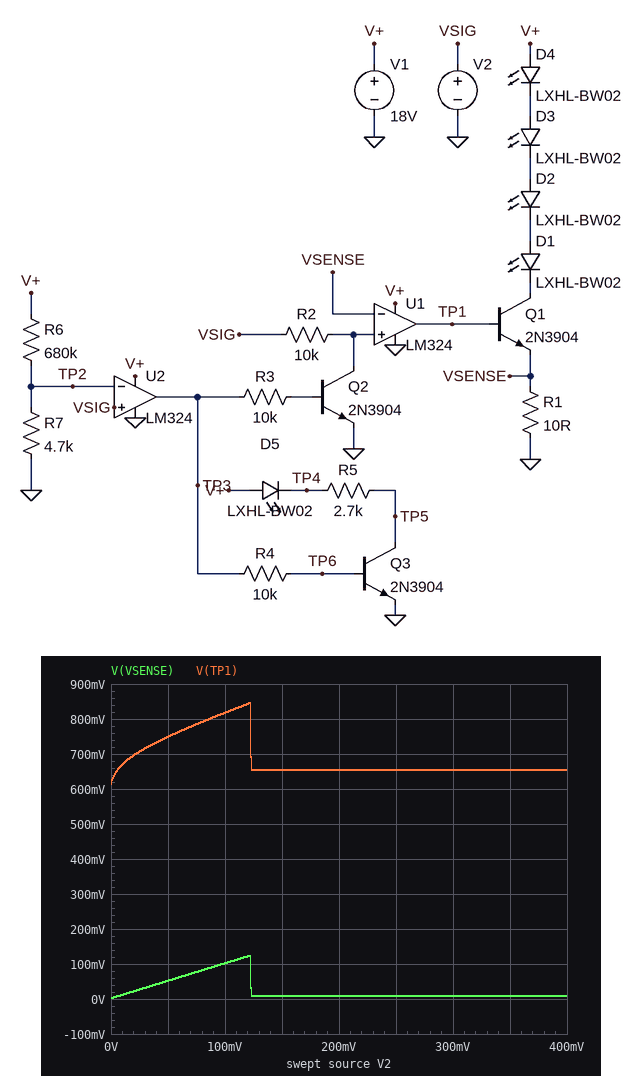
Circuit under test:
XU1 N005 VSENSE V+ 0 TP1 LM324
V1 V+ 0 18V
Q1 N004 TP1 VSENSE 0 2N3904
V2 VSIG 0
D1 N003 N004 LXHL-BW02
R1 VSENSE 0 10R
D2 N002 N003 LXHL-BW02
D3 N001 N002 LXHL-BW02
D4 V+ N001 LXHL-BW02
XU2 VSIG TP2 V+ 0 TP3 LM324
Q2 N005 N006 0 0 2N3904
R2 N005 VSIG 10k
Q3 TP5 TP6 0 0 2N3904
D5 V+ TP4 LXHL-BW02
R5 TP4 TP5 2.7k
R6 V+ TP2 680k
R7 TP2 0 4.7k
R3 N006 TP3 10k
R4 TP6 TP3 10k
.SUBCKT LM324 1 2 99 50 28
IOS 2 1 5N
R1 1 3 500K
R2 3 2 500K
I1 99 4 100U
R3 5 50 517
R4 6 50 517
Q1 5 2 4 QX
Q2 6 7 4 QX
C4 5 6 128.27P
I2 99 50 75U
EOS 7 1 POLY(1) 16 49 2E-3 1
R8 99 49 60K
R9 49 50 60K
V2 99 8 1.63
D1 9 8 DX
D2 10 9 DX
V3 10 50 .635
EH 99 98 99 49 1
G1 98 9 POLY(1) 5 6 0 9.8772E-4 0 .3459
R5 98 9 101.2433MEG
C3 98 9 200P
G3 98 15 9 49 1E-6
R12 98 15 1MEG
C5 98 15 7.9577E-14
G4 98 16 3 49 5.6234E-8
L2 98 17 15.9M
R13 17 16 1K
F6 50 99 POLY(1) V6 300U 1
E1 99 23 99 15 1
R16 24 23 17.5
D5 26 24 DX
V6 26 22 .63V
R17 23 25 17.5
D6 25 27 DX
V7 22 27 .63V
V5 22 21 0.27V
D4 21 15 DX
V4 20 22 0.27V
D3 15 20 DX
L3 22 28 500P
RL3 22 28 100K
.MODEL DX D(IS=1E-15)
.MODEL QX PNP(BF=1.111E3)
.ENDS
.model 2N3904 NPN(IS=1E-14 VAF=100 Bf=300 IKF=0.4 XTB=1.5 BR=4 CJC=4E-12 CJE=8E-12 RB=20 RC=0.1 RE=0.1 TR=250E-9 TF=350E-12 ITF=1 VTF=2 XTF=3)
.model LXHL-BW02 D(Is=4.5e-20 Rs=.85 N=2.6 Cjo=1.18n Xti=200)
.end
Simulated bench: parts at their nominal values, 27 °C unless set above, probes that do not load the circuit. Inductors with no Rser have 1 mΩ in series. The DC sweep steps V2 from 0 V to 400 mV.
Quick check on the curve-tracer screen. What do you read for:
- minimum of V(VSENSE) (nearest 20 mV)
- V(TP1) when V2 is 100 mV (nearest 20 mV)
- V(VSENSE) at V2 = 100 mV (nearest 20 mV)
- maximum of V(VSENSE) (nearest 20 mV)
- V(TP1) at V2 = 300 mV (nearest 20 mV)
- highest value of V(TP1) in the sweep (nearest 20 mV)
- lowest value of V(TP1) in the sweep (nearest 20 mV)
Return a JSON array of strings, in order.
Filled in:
["0 V", "820 mV", "100 mV", "120 mV", "660 mV", "840 mV", "620 mV"]
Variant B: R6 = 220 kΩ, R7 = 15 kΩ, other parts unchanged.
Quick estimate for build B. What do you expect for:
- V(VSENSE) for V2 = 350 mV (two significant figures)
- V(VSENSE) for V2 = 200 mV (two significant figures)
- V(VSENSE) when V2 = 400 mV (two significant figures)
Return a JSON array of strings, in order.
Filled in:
["350 mV", "200 mV", "400 mV"]
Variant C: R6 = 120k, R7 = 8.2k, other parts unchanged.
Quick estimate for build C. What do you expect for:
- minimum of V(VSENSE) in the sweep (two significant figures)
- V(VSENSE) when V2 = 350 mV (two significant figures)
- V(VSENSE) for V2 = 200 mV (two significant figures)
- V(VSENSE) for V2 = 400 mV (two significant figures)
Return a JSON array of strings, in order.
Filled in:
["2.1 mV", "350 mV", "200 mV", "400 mV"]
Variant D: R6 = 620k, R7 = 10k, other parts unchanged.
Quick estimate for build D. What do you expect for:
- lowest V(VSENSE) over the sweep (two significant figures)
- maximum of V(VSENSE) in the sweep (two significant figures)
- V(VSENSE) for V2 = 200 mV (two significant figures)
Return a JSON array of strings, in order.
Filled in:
["2.1 mV", "290 mV", "200 mV"]
